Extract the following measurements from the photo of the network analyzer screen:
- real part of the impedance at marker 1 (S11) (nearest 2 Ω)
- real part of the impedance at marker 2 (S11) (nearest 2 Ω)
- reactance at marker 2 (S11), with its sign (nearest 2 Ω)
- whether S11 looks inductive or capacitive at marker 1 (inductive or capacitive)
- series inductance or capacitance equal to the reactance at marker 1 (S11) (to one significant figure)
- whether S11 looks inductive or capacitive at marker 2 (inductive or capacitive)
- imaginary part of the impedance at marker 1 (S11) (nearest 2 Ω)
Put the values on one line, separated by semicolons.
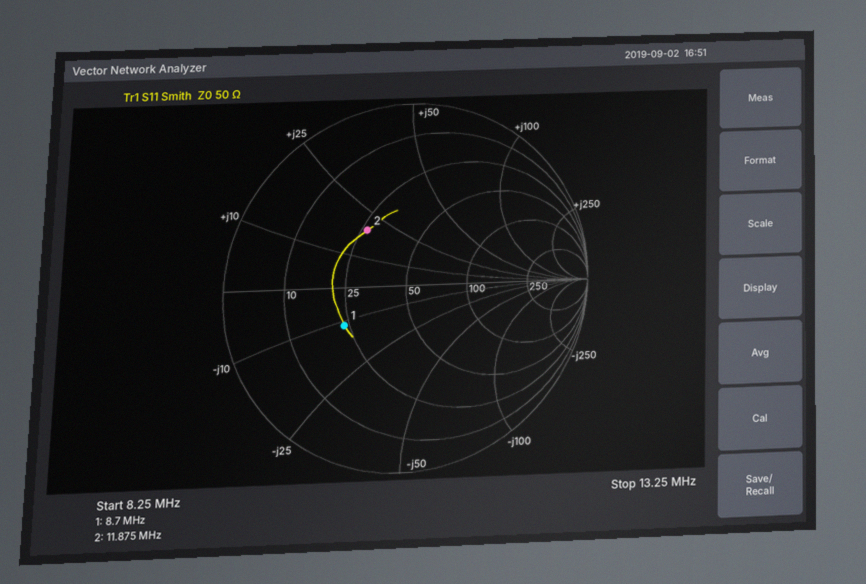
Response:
24 Ω; 26 Ω; +20 Ω; capacitive; 2 nF; inductive; -12 Ω
